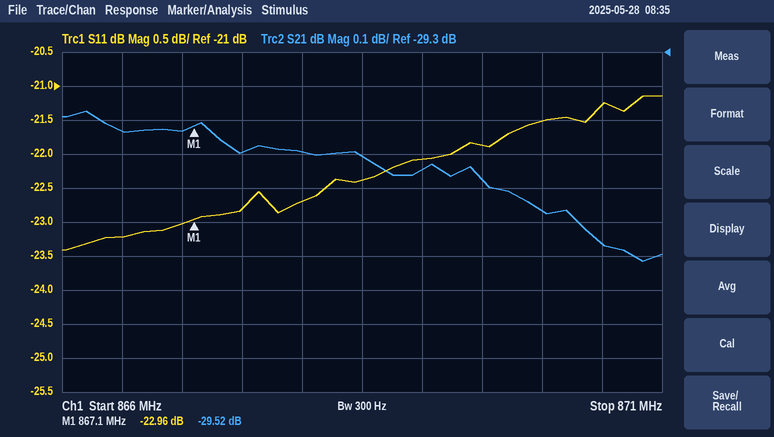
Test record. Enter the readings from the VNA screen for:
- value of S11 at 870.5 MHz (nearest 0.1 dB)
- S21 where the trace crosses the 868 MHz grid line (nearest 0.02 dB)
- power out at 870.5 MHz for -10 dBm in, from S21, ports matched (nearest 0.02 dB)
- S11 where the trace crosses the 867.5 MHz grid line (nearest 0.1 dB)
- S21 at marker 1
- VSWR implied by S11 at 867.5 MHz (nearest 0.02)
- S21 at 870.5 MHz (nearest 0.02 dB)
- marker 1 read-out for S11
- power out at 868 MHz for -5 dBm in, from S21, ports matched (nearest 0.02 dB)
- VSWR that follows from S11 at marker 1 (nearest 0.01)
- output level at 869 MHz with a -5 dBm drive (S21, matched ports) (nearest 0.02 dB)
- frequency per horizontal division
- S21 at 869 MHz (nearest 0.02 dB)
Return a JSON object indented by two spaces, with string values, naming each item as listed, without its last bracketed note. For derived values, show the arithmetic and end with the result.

{
  "value of S11 at 870.5 MHz": "-21.3 dB",
  "S21 where the trace crosses the 868 MHz grid line": "-29.60 dB",
  "power out at 870.5 MHz for -10 dBm in, from S21, ports matched": "-10 dBm + (-29.86 dB) = -39.86 dBm",
  "S11 where the trace crosses the 867.5 MHz grid line": "-22.8 dB",
  "S21 at marker 1": "-29.52 dB",
  "VSWR implied by S11 at 867.5 MHz": "|Γ| = 10^(-22.8/20) = 0.0724; VSWR = (1 + 0.0724)/(1 − 0.0724) ≈ 1.16",
  "S21 at 870.5 MHz": "-29.86 dB",
  "marker 1 read-out for S11": "-22.96 dB",
  "power out at 868 MHz for -5 dBm in, from S21, ports matched": "-5 dBm + (-29.60 dB) = -34.60 dBm",
  "VSWR that follows from S11 at marker 1": "(1 + 0.0711)/(1 − 0.0711) ≈ 1.15",
  "output level at 869 MHz with a -5 dBm drive (S21, matched ports)": "-5 dBm + (-29.64 dB) = -34.64 dBm",
  "frequency per horizontal division": "500 kHz",
  "S21 at 869 MHz": "-29.64 dB"
}
